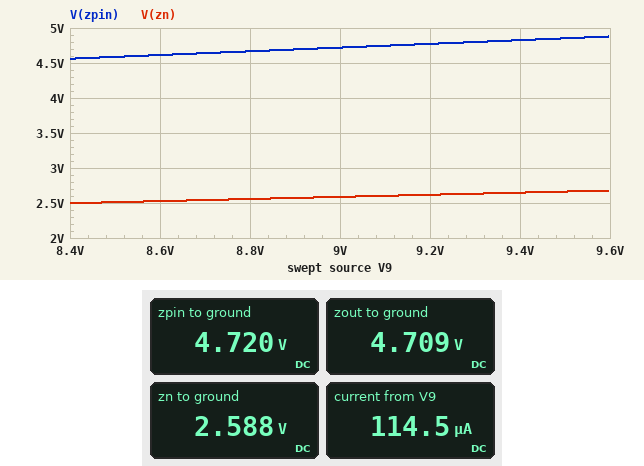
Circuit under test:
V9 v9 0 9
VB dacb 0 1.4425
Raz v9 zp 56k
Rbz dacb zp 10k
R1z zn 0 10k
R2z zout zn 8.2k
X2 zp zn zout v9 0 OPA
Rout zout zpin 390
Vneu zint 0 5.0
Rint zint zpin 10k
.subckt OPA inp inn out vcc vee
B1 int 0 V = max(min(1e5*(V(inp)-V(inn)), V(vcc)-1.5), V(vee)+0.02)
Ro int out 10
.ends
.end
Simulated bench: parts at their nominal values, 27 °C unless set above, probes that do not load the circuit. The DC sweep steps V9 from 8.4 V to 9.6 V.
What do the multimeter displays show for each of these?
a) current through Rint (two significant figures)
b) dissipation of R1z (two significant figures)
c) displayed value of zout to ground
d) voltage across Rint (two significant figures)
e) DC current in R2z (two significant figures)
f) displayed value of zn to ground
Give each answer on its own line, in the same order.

28 µA
670 µW
4.709 V
280 mV
260 µA
2.588 V
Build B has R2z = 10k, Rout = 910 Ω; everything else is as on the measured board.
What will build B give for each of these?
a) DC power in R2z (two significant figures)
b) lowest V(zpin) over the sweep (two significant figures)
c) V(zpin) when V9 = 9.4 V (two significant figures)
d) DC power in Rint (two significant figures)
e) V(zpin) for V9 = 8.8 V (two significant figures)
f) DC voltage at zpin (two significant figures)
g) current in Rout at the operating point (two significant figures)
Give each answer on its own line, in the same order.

670 µW
5.0 V
5.3 V
2.6 µW
5.1 V
5.2 V
16 µA
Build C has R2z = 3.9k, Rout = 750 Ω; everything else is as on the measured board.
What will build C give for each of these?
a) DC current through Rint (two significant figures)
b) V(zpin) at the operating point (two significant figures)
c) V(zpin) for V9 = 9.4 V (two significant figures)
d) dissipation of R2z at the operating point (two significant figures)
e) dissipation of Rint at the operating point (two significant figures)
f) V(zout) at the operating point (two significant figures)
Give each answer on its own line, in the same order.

130 µA
3.7 V
3.8 V
260 µW
170 µW
3.6 V
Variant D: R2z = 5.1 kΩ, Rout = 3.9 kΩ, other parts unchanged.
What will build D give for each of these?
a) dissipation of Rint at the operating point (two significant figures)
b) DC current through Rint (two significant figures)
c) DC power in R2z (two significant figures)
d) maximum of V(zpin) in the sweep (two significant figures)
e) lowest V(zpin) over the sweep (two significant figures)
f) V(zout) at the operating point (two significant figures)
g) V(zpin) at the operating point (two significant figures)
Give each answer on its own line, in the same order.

62 µW
79 µA
340 µW
4.3 V
4.1 V
3.9 V
4.2 V
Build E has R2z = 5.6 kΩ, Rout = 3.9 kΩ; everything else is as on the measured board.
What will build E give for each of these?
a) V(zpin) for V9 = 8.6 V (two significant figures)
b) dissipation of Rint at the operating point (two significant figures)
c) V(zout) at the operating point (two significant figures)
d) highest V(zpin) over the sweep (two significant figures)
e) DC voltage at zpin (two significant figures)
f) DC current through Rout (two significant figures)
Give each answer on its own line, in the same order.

4.2 V
48 µW
4.0 V
4.4 V
4.3 V
69 µA
